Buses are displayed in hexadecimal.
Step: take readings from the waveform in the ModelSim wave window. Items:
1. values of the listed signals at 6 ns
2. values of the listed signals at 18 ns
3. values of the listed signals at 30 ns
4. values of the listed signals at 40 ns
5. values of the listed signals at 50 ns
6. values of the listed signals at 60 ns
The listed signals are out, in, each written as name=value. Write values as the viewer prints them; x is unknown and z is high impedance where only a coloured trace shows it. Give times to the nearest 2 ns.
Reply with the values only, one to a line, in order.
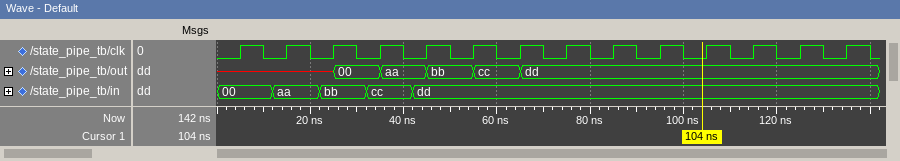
out=x, in=00
out=x, in=aa
out=00, in=bb
out=aa, in=cc
out=bb, in=dd
out=cc, in=dd
